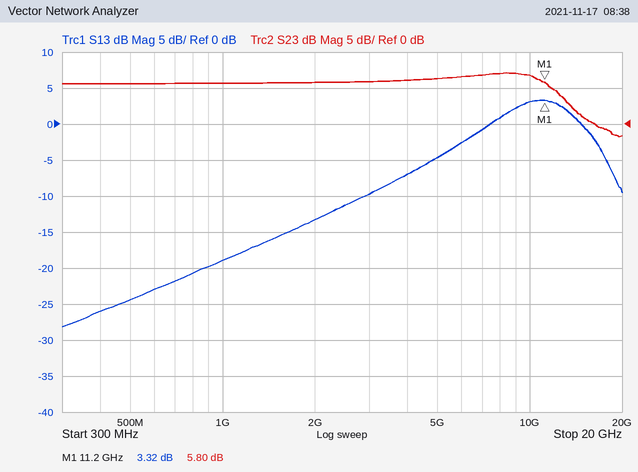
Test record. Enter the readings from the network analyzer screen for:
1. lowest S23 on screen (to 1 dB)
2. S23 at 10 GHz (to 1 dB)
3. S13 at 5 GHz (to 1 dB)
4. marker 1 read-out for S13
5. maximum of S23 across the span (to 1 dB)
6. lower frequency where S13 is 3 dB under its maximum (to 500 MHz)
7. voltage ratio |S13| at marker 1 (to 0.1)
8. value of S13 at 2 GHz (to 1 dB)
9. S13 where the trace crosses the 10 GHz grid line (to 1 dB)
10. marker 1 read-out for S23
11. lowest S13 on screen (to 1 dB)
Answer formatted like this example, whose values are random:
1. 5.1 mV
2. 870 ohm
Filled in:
1. -2 dB
2. 7 dB
3. -5 dB
4. 3.32 dB
5. 7 dB
6. 7.5 GHz
7. 1.5
8. -13 dB
9. 3 dB
10. 5.80 dB
11. -28 dB
